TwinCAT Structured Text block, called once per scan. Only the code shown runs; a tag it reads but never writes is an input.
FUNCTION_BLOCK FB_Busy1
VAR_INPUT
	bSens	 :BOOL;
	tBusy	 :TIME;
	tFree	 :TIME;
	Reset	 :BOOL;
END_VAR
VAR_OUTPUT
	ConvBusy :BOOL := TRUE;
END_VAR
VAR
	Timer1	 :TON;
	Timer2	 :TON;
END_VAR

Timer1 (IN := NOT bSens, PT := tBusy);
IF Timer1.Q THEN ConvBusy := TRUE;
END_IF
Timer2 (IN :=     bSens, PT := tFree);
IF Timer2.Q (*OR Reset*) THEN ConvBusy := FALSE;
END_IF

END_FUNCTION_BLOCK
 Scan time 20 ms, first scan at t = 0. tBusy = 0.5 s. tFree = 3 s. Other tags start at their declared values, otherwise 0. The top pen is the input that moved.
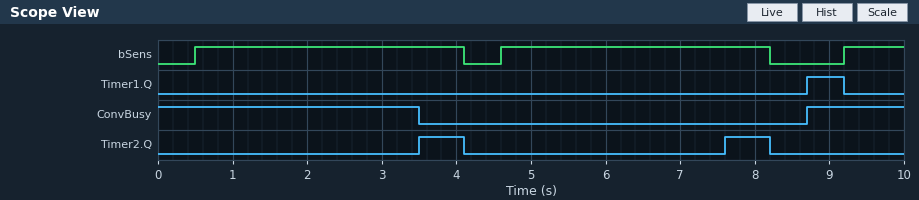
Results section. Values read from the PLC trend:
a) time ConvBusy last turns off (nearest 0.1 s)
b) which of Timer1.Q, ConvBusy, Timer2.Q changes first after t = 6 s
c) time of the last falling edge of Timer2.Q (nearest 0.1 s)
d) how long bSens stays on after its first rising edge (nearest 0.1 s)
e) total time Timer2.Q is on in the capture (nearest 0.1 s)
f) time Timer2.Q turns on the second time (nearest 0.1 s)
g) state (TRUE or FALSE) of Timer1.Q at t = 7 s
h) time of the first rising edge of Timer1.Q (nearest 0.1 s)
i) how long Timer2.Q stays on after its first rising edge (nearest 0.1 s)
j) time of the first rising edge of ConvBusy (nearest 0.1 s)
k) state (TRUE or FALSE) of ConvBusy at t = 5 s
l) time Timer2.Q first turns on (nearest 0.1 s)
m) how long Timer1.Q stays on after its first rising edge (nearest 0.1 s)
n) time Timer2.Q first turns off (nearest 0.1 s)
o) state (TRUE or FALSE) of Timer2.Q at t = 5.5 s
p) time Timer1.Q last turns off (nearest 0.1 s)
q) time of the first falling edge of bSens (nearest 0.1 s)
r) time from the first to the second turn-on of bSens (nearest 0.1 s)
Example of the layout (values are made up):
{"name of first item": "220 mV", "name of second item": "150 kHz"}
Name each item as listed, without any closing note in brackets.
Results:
{"time ConvBusy last turns off": "3.5 s", "which of Timer1.Q, ConvBusy, Timer2.Q changes first after t = 6 s": "Timer2.Q", "time of the last falling edge of Timer2.Q": "8.2 s", "how long bSens stays on after its first rising edge": "3.6 s", "total time Timer2.Q is on in the capture": "1.2 s", "time Timer2.Q turns on the second time": "7.6 s", "state (TRUE or FALSE) of Timer1.Q at t = 7 s": "FALSE", "time of the first rising edge of Timer1.Q": "8.7 s", "how long Timer2.Q stays on after its first rising edge": "0.6 s", "time of the first rising edge of ConvBusy": "8.7 s", "state (TRUE or FALSE) of ConvBusy at t = 5 s": "FALSE", "time Timer2.Q first turns on": "3.5 s", "how long Timer1.Q stays on after its first rising edge": "0.5 s", "time Timer2.Q first turns off": "4.1 s", "state (TRUE or FALSE) of Timer2.Q at t = 5.5 s": "FALSE", "time Timer1.Q last turns off": "9.2 s", "time of the first falling edge of bSens": "4.1 s", "time from the first to the second turn-on of bSens": "4.1 s"}
